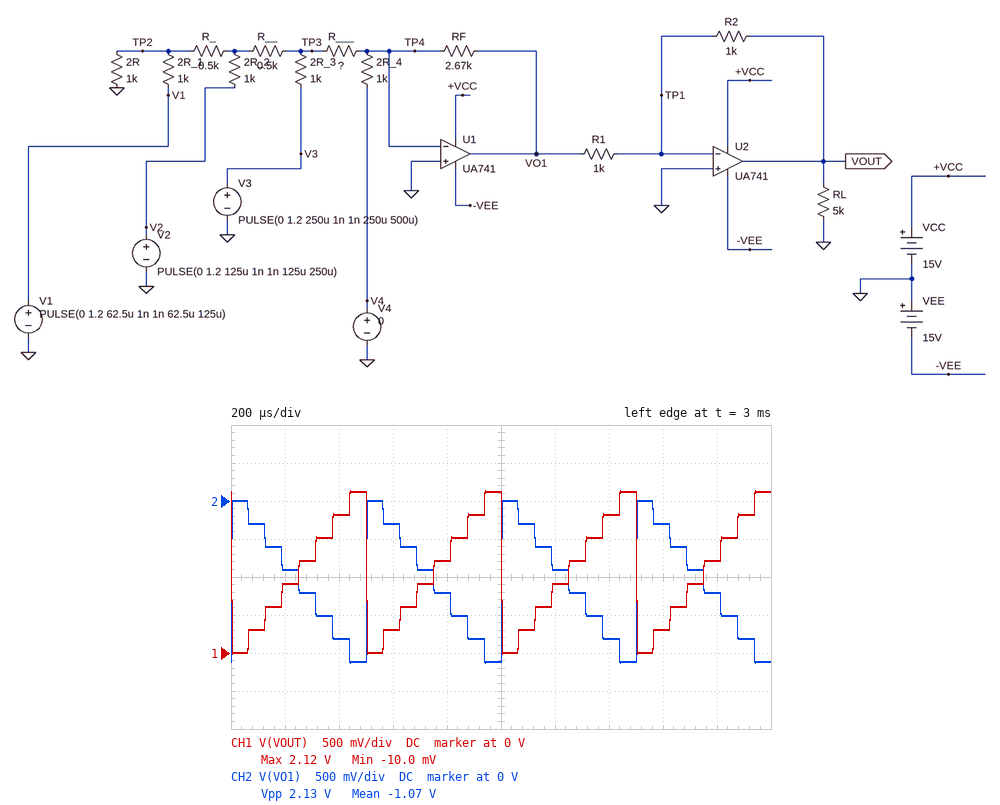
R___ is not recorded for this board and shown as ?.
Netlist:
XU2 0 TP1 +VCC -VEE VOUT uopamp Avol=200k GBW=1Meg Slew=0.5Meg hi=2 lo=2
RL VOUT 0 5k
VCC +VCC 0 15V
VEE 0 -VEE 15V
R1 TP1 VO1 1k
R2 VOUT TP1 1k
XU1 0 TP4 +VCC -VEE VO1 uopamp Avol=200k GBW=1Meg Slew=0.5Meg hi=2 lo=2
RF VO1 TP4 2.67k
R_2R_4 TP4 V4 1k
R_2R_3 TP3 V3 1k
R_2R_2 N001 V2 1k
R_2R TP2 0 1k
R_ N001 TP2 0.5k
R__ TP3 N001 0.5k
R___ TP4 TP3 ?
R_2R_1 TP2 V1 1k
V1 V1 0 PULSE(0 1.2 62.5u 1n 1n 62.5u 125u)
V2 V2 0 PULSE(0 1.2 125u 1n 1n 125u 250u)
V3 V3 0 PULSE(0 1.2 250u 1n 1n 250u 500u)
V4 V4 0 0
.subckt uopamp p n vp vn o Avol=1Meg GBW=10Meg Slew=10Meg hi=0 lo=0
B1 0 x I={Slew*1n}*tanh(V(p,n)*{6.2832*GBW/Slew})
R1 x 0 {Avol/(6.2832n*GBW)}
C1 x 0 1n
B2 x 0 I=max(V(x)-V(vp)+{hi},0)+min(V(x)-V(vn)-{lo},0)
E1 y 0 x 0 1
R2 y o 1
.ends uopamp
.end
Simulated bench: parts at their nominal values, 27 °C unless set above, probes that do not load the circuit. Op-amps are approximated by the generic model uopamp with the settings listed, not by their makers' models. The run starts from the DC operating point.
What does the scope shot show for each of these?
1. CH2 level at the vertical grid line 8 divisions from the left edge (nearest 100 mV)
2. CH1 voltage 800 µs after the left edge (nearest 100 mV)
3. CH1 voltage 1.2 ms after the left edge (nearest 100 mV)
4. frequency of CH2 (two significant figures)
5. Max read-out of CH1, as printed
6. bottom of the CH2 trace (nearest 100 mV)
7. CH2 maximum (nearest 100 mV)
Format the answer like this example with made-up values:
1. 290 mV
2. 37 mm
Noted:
1. -300 mV
2. 1.2 V
3. 900 mV
4. 2.0 kHz
5. 2.12 V
6. -2.1 V
7. 0 V
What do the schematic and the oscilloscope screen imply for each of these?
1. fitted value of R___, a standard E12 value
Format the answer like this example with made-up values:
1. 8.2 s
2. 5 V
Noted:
1. 820 Ω
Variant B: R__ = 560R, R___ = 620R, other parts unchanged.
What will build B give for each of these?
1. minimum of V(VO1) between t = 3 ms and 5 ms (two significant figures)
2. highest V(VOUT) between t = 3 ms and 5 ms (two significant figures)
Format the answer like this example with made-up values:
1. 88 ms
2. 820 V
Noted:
1. -2.5 V
2. 2.5 V
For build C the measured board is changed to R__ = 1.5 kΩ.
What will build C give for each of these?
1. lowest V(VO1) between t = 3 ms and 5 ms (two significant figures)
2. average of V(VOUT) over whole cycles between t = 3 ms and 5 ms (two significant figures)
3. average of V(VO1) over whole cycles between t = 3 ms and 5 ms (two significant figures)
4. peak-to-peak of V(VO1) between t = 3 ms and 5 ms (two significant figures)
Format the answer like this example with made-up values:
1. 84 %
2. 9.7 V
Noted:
1. -2.0 V
2. 990 mV
3. -990 mV
4. 2.0 V
